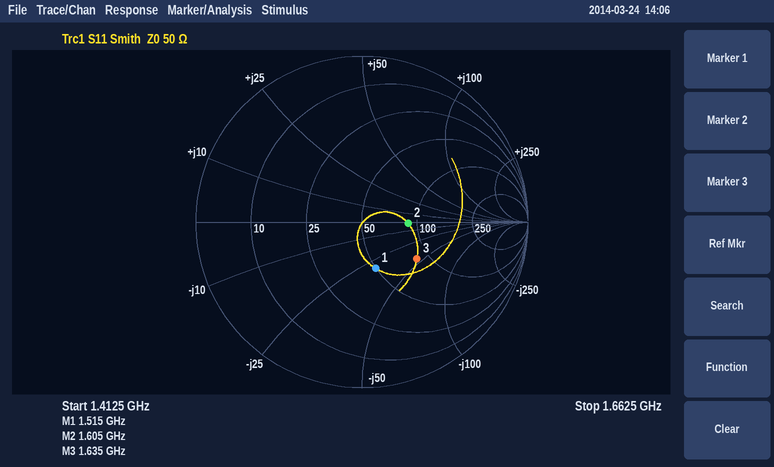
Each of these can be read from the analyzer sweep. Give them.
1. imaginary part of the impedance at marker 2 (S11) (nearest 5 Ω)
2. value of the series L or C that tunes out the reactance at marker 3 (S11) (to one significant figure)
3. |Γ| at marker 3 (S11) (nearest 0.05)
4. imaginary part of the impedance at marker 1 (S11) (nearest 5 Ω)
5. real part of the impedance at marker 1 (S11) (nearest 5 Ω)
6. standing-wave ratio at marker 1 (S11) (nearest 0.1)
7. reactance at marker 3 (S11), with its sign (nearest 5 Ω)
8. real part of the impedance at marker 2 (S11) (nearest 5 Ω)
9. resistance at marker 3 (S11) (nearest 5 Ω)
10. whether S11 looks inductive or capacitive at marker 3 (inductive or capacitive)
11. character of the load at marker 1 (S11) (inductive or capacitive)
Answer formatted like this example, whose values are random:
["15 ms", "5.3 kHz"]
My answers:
["0 Ω", "4 nH", "0.40", "-30 Ω", "50 Ω", "1.8", "-45 Ω", "90 Ω", "85 Ω", "capacitive", "capacitive"]
